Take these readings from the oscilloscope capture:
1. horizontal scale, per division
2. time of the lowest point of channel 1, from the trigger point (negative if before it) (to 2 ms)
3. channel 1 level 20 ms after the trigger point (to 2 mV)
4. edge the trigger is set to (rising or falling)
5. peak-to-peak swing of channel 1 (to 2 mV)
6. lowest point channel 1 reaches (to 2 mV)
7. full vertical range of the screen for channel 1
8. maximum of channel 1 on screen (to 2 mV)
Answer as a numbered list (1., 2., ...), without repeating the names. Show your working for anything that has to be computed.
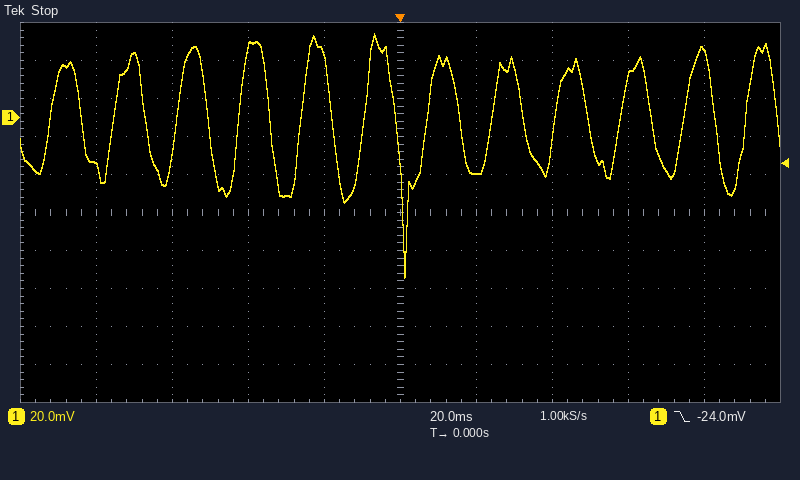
1. 20 ms
2. +2 ms
3. -30 mV
4. falling
5. 44 mV − (-84 mV) = 128 mV
6. -84 mV
7. 200 mV
8. 44 mV
